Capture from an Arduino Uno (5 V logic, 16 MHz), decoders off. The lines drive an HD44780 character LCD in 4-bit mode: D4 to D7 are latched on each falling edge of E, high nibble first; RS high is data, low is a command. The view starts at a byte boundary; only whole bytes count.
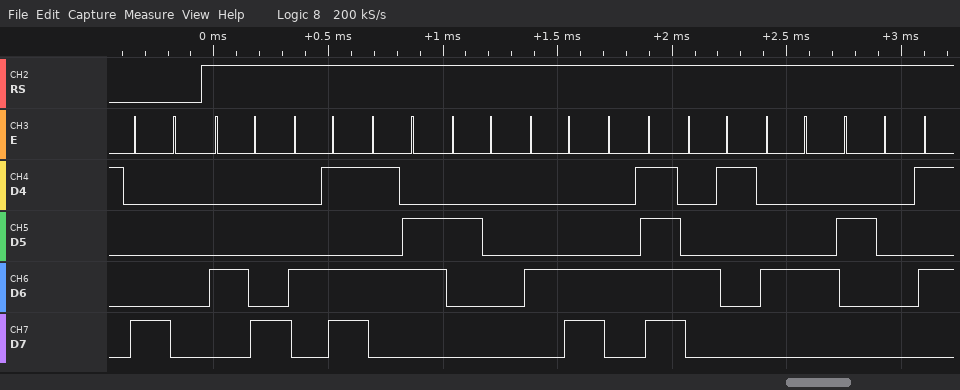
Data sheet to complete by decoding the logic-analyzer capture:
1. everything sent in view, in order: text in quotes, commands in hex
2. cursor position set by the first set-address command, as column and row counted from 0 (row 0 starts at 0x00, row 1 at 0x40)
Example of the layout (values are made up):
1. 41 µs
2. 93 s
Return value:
1. 0x80 "HMV LOAD "
2. column 0, row 0
